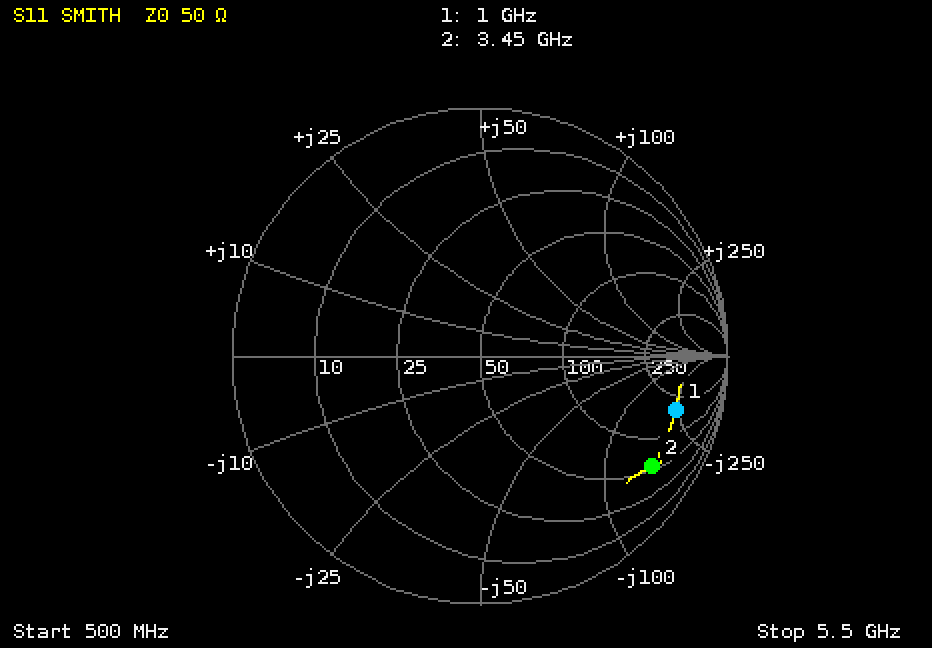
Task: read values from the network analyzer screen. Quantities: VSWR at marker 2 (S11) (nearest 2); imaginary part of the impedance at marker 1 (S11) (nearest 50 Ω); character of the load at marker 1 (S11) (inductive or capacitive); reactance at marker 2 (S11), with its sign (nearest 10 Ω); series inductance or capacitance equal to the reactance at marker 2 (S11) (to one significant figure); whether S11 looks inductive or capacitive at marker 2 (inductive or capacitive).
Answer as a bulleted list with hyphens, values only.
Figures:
- 10
- -250 Ω
- capacitive
- -150 Ω
- 300 fF
- capacitive
